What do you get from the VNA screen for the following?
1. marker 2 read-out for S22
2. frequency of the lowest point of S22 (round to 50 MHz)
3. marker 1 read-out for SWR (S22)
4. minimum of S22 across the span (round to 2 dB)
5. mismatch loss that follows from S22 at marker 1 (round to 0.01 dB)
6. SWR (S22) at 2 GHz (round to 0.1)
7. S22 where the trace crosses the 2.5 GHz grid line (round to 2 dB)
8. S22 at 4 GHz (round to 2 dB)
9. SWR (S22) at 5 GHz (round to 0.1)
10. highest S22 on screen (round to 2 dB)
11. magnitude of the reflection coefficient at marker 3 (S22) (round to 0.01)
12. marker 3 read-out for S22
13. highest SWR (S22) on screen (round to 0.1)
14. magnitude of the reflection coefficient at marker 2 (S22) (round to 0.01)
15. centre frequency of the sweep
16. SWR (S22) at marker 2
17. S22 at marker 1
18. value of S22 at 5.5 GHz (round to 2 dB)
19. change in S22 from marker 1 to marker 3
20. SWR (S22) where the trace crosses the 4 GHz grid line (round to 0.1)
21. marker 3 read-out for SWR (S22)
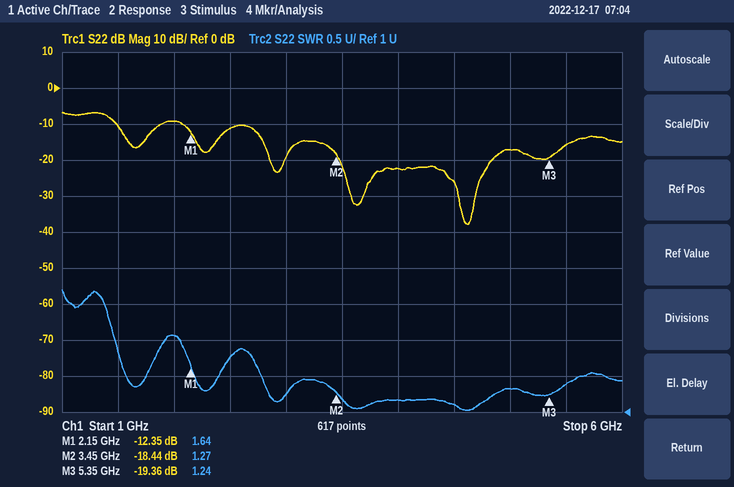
-18.44 dB
4.60 GHz
1.64
-38 dB
0.26 dB
2.1
-12 dB
-22 dB
1.3
-6 dB
0.11
-19.36 dB
2.7
0.12
3.5 GHz
1.27
-12.35 dB
-16 dB
-7.01 dB
1.2
1.24
